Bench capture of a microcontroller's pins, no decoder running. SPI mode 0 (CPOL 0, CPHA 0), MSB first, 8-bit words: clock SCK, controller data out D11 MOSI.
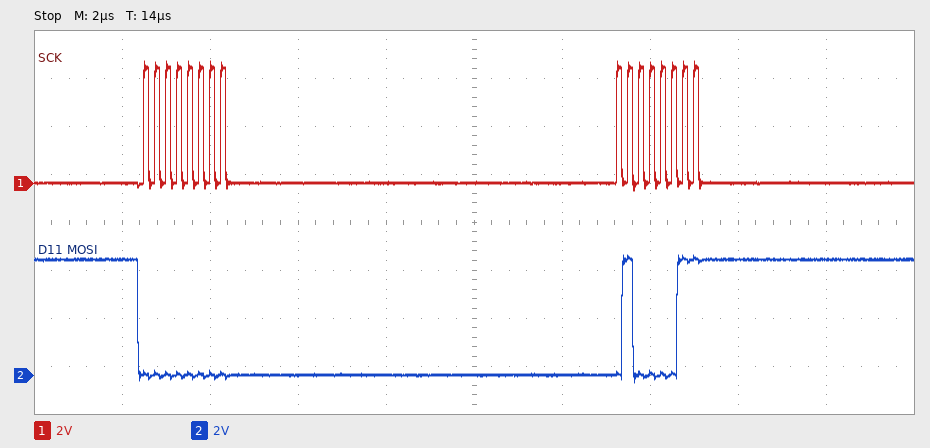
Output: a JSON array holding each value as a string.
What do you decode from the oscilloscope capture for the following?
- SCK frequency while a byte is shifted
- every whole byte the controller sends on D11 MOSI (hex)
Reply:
["4 MHz", "0x00 0x43"]
